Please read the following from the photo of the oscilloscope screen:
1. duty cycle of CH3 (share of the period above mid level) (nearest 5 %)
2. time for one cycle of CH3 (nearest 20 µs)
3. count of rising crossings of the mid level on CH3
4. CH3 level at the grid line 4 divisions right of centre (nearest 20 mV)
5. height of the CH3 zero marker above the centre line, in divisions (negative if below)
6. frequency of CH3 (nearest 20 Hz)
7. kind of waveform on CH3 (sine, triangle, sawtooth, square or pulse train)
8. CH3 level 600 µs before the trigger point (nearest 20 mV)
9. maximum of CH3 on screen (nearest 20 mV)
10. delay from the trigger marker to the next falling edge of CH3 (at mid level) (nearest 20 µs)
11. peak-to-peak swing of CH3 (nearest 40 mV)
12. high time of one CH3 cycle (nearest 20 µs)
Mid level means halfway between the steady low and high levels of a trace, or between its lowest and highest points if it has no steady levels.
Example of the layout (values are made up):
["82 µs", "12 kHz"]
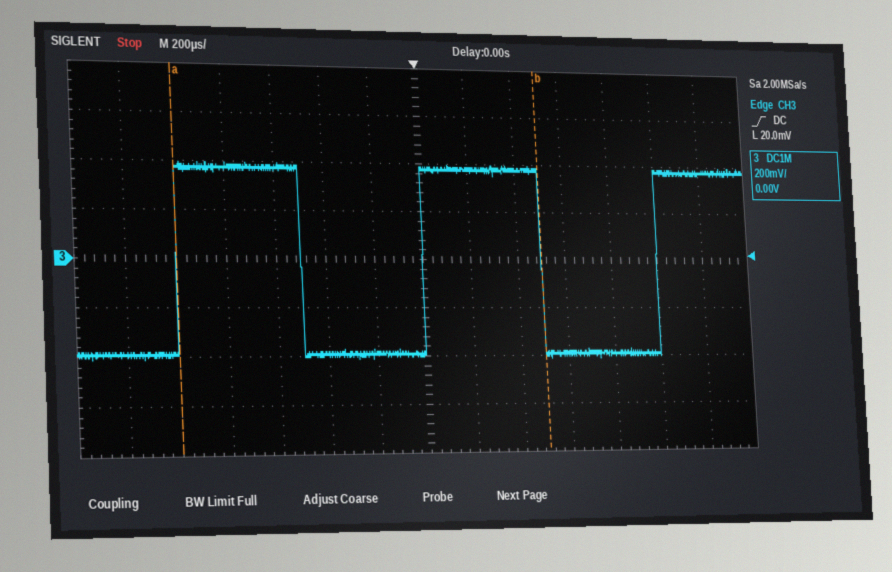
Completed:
["50 %", "1.00 ms", "3", "-400 mV", "0.0 div", "1.00 kHz", "square", "380 mV", "400 mV", "500 µs", "800 mV", "500 µs"]
